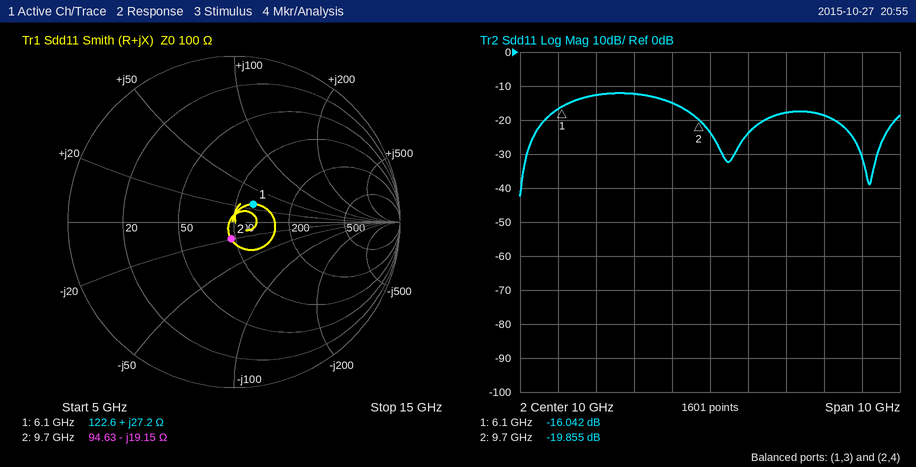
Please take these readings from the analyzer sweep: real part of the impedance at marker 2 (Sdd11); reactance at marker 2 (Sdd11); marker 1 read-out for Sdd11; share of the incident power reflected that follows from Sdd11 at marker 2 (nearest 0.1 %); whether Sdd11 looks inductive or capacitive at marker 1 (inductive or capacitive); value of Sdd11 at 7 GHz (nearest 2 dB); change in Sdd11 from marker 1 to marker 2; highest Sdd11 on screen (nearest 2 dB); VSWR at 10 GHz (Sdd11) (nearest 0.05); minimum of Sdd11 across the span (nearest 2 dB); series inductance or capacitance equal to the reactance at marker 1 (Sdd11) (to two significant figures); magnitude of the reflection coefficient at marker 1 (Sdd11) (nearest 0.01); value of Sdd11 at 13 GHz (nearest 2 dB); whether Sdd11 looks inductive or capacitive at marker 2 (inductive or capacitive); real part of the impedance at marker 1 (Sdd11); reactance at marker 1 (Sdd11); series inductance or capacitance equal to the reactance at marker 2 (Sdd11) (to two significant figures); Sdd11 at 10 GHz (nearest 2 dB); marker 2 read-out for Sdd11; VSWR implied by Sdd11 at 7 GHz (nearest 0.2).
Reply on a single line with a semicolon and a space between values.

94.63 Ω; -19.15 Ω; -16.042 dB; 1.0 %; inductive; -12 dB; -3.813 dB; -12 dB; 1.15; -42 dB; 710 pH; 0.16; -18 dB; capacitive; 122.6 Ω; +27.2 Ω; 860 fF; -24 dB; -19.855 dB; 1.6
